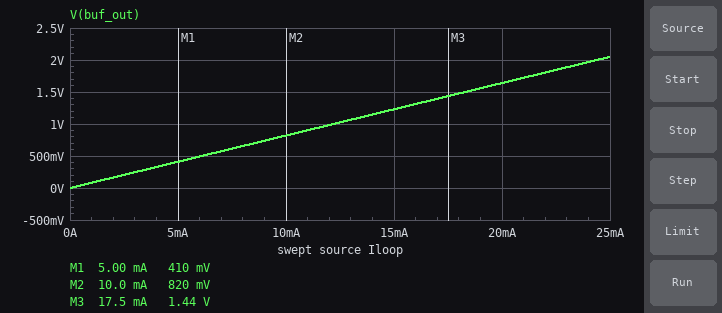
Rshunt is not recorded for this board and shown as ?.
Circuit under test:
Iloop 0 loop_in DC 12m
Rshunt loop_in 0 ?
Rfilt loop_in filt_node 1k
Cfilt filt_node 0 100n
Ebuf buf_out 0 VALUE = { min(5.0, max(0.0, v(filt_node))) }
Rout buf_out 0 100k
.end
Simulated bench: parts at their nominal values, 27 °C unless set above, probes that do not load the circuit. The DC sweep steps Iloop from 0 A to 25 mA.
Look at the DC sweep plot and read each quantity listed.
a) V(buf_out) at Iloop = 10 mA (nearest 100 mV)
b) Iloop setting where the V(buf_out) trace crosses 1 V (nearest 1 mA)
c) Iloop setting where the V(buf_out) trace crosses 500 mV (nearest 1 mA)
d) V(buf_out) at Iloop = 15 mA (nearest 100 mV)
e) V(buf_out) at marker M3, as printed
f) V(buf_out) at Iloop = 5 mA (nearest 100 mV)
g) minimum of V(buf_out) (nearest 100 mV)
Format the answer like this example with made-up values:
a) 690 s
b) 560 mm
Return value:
a) 800 mV
b) 12 mA
c) 6 mA
d) 1.2 V
e) 1.44 V
f) 400 mV
g) 0 V
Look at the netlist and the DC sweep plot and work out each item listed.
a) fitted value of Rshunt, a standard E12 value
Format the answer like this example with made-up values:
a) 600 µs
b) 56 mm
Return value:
a) 82 Ω
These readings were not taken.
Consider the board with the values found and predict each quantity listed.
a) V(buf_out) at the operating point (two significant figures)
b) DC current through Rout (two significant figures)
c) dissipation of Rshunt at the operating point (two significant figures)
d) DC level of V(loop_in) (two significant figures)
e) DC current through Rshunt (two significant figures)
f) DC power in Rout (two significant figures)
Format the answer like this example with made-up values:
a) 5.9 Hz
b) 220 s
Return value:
a) 980 mV
b) 9.8 µA
c) 12 mW
d) 980 mV
e) 12 mA
f) 9.7 µW
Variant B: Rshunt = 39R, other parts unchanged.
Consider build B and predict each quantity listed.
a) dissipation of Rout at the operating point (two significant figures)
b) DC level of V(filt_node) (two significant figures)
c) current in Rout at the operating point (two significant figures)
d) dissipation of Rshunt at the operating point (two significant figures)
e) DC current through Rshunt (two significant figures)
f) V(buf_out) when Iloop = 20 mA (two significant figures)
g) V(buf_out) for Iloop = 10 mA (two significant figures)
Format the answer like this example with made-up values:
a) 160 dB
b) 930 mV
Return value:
a) 2.2 µW
b) 470 mV
c) 4.7 µA
d) 5.6 mW
e) 12 mA
f) 780 mV
g) 390 mV
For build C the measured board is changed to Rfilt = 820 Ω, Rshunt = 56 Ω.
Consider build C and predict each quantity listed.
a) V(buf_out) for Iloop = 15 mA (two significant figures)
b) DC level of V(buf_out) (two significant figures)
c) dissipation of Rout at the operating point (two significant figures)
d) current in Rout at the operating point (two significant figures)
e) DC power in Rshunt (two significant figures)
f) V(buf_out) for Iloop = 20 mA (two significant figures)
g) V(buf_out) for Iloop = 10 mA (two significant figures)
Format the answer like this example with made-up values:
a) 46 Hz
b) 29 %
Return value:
a) 840 mV
b) 670 mV
c) 4.5 µW
d) 6.7 µA
e) 8.1 mW
f) 1.1 V
g) 560 mV
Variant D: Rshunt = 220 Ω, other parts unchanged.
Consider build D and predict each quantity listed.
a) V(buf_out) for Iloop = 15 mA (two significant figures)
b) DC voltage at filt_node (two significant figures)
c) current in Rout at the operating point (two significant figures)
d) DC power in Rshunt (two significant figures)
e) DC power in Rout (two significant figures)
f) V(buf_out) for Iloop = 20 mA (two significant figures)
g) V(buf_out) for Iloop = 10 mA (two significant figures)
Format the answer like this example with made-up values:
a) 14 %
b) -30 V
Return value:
a) 3.3 V
b) 2.6 V
c) 26 µA
d) 32 mW
e) 70 µW
f) 4.4 V
g) 2.2 V
